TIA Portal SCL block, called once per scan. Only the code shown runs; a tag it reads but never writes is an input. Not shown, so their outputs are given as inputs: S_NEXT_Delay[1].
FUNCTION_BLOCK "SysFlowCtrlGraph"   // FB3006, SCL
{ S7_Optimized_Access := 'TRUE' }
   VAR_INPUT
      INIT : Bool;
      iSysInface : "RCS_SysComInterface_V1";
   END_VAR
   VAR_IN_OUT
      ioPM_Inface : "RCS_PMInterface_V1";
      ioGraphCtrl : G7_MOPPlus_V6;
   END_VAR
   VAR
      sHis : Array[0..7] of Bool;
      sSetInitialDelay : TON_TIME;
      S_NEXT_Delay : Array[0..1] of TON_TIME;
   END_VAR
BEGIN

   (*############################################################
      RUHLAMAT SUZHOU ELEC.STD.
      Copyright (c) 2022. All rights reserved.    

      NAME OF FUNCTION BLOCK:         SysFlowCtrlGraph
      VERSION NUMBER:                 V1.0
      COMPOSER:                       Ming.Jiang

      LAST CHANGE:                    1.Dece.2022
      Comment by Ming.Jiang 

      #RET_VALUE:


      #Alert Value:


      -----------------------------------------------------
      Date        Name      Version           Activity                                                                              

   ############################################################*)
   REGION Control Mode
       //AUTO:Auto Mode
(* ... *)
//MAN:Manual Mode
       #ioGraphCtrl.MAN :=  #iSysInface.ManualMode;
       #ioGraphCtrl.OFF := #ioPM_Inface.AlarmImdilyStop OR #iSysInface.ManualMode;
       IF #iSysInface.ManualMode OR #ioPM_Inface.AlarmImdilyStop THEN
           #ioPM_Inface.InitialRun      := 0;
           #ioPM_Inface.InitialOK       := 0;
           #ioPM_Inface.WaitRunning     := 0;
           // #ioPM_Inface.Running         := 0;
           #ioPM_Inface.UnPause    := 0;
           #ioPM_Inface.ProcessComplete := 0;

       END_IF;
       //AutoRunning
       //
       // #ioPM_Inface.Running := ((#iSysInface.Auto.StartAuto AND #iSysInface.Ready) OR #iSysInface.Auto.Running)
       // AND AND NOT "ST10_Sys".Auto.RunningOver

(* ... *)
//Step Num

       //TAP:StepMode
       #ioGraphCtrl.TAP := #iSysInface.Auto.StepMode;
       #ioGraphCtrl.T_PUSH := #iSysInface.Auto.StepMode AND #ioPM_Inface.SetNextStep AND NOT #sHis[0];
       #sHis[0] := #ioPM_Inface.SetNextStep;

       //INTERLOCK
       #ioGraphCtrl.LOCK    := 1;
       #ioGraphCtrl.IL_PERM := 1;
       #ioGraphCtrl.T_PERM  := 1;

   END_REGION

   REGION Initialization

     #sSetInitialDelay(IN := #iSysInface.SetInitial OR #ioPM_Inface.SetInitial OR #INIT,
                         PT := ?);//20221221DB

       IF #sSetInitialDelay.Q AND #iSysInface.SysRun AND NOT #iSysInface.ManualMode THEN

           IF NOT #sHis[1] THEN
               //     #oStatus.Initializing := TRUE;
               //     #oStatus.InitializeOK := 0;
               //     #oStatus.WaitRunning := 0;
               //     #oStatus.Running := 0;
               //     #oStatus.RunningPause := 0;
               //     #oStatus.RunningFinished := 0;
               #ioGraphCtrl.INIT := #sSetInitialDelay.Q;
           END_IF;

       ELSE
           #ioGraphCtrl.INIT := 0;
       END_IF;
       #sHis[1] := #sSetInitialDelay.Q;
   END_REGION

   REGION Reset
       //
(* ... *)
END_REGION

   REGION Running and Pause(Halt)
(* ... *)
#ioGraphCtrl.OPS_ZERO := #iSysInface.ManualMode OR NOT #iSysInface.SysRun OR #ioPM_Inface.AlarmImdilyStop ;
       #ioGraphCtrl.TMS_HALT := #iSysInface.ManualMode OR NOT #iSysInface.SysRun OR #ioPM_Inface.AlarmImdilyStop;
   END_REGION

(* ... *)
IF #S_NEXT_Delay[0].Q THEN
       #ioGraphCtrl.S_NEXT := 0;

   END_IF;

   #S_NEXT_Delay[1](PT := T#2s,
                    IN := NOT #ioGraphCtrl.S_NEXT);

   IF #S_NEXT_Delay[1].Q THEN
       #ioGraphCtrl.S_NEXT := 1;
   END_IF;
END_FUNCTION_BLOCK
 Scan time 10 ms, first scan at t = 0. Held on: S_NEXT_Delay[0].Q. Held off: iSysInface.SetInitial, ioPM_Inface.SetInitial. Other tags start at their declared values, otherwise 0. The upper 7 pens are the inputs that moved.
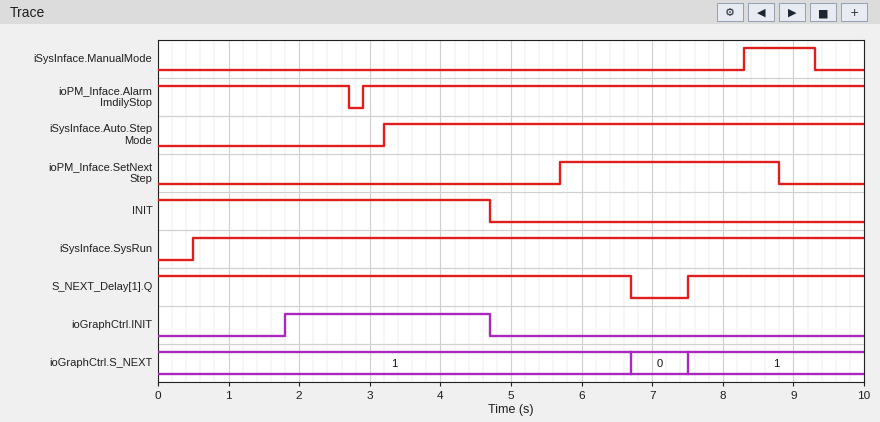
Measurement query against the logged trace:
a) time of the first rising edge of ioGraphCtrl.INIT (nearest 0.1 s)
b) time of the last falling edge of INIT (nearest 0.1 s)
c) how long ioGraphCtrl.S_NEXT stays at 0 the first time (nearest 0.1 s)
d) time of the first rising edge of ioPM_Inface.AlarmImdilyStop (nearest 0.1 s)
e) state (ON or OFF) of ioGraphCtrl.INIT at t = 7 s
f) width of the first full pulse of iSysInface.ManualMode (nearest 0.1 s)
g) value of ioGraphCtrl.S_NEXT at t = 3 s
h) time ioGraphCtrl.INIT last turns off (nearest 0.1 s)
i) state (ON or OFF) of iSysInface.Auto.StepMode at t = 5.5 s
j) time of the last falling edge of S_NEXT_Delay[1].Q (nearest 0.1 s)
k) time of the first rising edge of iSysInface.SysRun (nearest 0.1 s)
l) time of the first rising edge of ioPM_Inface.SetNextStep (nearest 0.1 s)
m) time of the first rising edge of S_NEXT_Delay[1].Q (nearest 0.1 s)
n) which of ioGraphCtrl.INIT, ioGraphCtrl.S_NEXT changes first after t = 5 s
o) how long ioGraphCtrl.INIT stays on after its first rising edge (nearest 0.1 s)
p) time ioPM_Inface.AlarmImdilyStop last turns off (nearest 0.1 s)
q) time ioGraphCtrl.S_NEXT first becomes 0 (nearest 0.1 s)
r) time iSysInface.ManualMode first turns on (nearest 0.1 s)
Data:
1.8 s
4.7 s
0.8 s
2.9 s
OFF
1.0 s
1
4.7 s
ON
6.7 s
0.5 s
5.7 s
7.5 s
ioGraphCtrl.S_NEXT
2.9 s
2.7 s
6.7 s
8.3 s
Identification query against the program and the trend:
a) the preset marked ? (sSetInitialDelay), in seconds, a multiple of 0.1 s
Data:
1.8 s
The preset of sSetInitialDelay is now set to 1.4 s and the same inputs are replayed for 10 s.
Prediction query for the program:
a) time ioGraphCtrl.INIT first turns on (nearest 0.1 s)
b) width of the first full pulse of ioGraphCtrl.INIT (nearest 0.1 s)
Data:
1.4 s
3.3 s
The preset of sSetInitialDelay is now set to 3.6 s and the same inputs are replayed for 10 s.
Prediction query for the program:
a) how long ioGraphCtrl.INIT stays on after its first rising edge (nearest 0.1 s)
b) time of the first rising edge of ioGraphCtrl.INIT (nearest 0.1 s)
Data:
1.1 s
3.6 s
